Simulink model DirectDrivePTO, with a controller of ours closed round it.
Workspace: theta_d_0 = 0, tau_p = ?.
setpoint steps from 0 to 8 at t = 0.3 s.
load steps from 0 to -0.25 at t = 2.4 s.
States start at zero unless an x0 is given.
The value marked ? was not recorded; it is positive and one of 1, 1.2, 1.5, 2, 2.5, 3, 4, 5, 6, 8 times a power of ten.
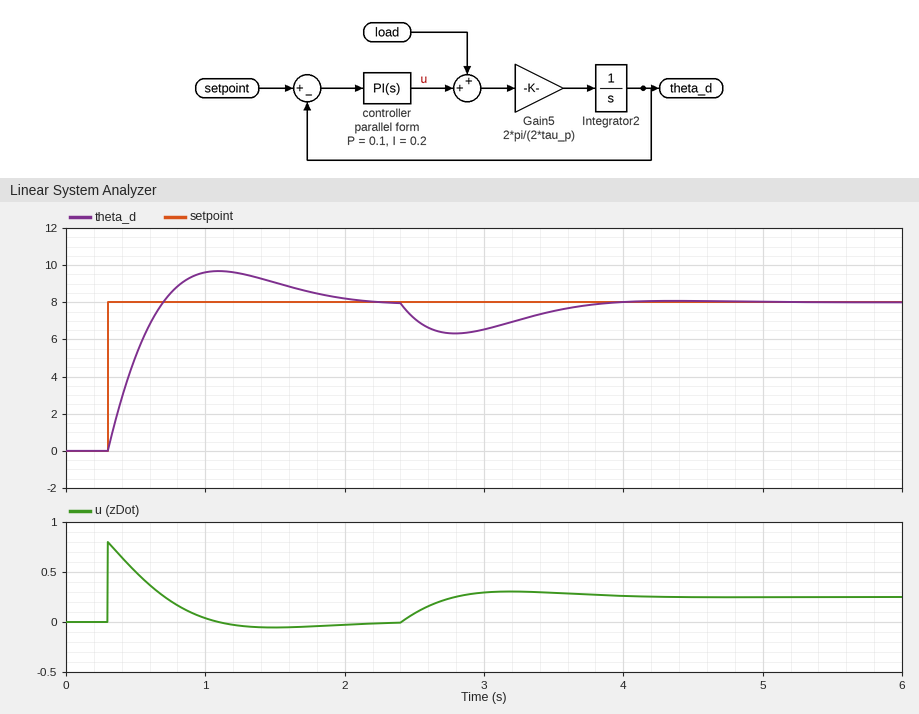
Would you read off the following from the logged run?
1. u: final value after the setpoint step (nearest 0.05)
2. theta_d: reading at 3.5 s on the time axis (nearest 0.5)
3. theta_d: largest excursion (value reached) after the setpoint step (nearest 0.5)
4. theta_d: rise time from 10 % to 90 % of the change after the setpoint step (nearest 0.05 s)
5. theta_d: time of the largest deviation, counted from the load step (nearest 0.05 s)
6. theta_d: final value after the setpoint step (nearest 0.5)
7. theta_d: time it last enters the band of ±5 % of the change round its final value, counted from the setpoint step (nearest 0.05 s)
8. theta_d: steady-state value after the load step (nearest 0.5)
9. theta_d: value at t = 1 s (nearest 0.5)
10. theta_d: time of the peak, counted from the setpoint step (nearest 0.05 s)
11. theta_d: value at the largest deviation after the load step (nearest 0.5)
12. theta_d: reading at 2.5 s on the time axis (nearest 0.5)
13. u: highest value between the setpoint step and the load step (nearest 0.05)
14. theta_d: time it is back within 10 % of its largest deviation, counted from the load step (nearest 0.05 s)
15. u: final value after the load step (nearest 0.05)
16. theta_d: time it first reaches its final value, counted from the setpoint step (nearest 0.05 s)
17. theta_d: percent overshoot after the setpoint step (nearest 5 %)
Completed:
0.00
7.5
9.5
0.30 s
0.40 s
8.0
1.55 s
8.0
9.5
0.80 s
6.5
7.0
0.80
1.35 s
0.25
0.40 s
20 %
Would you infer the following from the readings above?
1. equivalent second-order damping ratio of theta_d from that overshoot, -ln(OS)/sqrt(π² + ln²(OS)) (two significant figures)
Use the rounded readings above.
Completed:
0.46
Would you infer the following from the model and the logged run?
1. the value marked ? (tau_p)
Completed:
0.08
